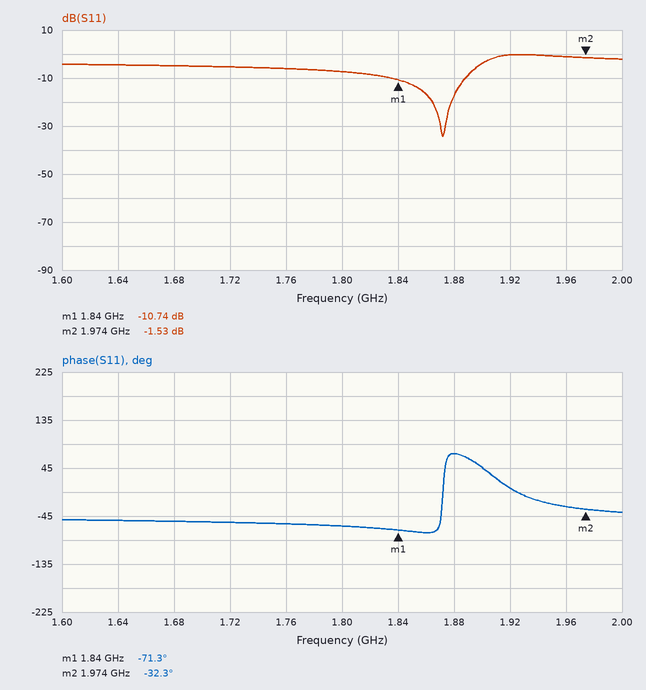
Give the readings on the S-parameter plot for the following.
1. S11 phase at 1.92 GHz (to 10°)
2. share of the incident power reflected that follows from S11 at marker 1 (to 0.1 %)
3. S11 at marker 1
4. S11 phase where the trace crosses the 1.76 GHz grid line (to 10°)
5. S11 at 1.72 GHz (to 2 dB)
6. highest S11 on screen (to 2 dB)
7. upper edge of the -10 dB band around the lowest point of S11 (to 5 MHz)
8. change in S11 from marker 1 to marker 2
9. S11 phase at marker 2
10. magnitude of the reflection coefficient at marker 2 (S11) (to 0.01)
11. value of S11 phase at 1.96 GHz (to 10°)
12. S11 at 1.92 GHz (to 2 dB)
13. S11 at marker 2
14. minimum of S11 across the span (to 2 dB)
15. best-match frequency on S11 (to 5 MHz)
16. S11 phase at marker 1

10°
8.4 %
-10.74 dB
-60°
-6 dB
0 dB
1.890 GHz
9.21 dB
-32.3°
0.84
-30°
0 dB
-1.53 dB
-34 dB
1.870 GHz
-71.3°
